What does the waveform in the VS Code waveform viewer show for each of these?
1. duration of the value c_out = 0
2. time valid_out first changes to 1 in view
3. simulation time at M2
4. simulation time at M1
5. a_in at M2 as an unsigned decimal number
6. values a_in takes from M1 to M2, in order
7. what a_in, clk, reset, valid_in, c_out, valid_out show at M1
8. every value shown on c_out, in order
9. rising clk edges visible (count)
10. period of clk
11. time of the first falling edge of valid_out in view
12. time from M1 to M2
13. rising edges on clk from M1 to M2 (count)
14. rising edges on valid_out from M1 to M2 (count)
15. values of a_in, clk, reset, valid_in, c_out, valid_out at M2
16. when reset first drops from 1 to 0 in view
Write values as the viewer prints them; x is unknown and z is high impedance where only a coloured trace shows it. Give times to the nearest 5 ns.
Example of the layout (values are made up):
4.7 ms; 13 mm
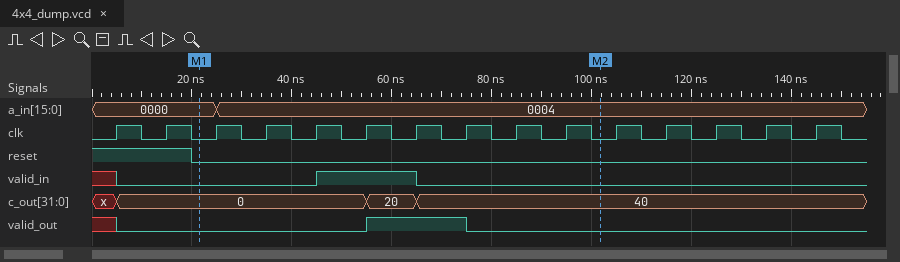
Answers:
50 ns; 55 ns; 100 ns; 20 ns; 4; 0000, 0004; a_in=0000, clk=0, reset=0, valid_in=0, c_out=0, valid_out=0; x, 0, 20, 40; 15; 10 ns; 75 ns; 80 ns; 8; 1; a_in=0004, clk=0, reset=0, valid_in=0, c_out=40, valid_out=0; 20 ns
